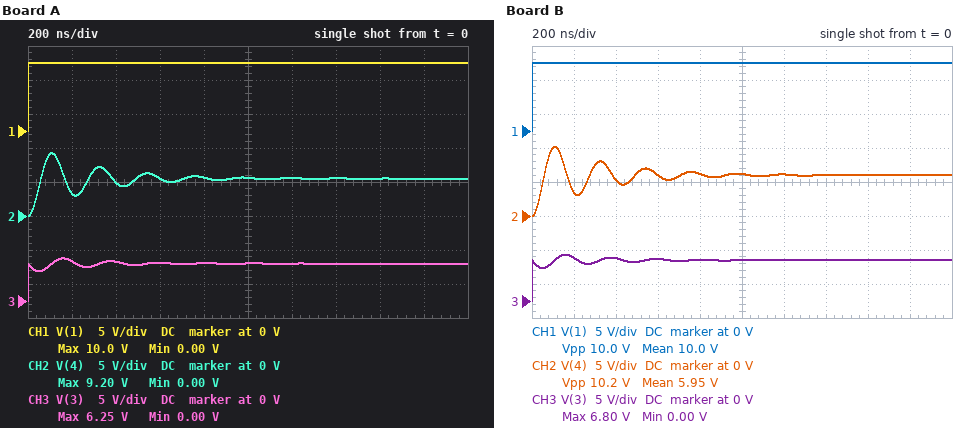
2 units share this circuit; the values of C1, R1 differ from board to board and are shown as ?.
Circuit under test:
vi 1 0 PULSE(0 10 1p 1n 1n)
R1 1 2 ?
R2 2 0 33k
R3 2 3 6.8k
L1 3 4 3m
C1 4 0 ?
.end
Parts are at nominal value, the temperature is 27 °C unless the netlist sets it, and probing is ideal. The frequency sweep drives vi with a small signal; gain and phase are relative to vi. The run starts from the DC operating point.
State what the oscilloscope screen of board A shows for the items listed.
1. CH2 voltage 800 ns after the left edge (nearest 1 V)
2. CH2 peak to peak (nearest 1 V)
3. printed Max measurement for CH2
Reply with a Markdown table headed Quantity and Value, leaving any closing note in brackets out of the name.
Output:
| Quantity | Value |
|---|---|
| CH2 voltage 800 ns after the left edge | 6 V |
| CH2 peak to peak | 9 V |
| printed Max measurement for CH2 | 9.20 V |
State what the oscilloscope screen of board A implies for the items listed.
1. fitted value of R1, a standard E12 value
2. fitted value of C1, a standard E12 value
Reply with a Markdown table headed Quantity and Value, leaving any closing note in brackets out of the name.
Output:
| Quantity | Value |
|---|---|
| fitted value of R1, a standard E12 value | 27 kΩ |
| fitted value of C1, a standard E12 value | 390 fF |
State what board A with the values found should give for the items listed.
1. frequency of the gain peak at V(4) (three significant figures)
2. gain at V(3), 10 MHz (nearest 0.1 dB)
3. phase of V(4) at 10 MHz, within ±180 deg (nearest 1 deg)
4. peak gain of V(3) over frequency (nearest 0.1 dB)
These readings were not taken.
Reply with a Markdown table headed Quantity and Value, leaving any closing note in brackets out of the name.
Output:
| Quantity | Value |
|---|---|
| frequency of the gain peak at V(4) | 4.58 MHz |
| gain at V(3), 10 MHz | -5.3 dB |
| phase of V(4) at 10 MHz, within ±180 deg | -172 deg |
| peak gain of V(3) over frequency | -5.2 dB |
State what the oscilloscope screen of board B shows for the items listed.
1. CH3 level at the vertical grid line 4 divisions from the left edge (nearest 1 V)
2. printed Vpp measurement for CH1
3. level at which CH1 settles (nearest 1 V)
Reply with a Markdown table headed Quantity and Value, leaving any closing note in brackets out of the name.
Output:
| Quantity | Value |
|---|---|
| CH3 level at the vertical grid line 4 divisions from the left edge | 6 V |
| printed Vpp measurement for CH1 | 10.0 V |
| level at which CH1 settles | 10 V |
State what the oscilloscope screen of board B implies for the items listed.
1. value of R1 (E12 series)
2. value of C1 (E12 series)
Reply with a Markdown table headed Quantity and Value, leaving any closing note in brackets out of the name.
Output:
| Quantity | Value |
|---|---|
| value of R1 | 22 kΩ |
| value of C1 | 390 fF |
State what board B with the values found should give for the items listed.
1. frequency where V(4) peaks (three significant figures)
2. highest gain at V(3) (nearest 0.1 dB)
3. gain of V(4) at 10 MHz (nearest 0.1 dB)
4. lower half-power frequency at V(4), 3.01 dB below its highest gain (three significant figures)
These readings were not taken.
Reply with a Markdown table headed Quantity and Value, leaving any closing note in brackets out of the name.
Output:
| Quantity | Value |
|---|---|
| frequency where V(4) peaks | 4.59 MHz |
| highest gain at V(3) | -4.4 dB |
| gain of V(4) at 10 MHz | -15.7 dB |
| lower half-power frequency at V(4), 3.01 dB below its highest gain | 4.02 MHz |
